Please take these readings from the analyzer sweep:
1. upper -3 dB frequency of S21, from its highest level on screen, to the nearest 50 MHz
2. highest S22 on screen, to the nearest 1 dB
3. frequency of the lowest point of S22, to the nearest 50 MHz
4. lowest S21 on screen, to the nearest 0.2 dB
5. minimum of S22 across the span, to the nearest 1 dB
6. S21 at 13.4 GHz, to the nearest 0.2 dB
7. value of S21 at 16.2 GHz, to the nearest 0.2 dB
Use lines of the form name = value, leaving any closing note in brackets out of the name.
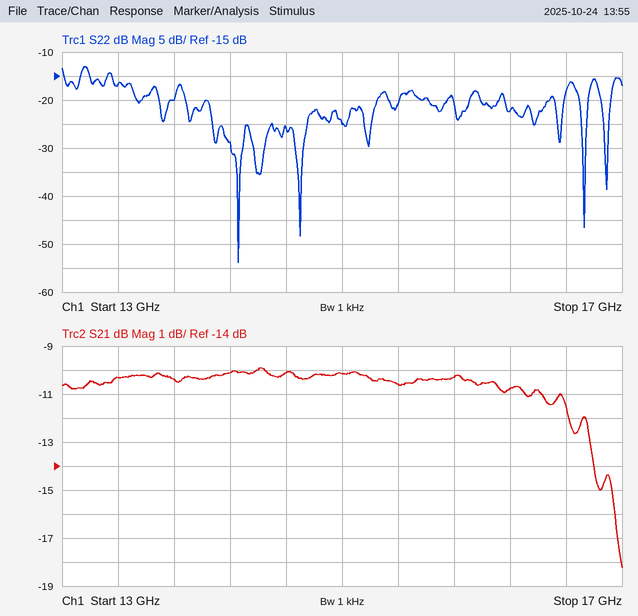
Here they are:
upper -3 dB frequency of S21, from its highest level on screen, to the nearest 50 MHz = 16.75 GHz
highest S22 on screen, to the nearest 1 dB = -13 dB
frequency of the lowest point of S22, to the nearest 50 MHz = 14.25 GHz
lowest S21 on screen, to the nearest 0.2 dB = -18.2 dB
minimum of S22 across the span, to the nearest 1 dB = -54 dB
S21 at 13.4 GHz, to the nearest 0.2 dB = -10.4 dB
value of S21 at 16.2 GHz, to the nearest 0.2 dB = -10.8 dB
